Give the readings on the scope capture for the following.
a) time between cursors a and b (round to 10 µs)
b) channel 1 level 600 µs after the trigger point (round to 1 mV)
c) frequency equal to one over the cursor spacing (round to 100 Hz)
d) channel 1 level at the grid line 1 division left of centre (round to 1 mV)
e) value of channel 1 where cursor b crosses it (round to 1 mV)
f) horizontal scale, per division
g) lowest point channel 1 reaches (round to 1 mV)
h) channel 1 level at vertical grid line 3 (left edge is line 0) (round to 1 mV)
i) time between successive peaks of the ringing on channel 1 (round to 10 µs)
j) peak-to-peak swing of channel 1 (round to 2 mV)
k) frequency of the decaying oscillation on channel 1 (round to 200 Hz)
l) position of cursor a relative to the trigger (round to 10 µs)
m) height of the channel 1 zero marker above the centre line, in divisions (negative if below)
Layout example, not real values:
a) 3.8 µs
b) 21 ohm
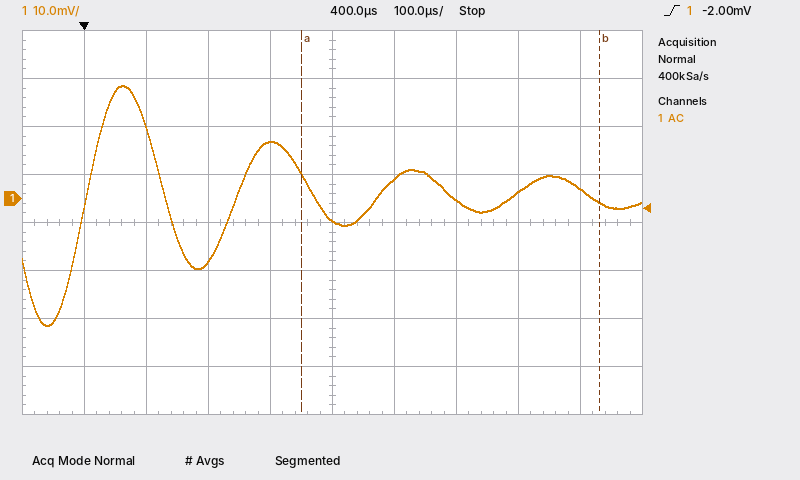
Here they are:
a) 480 µs
b) 0 mV
c) 2.1 kHz
d) 12 mV
e) -1 mV
f) 100 µs
g) -26 mV
h) -13 mV
i) 230 µs
j) 50 mV
k) 4.4 kHz
l) +350 µs
m) +0.5 div
